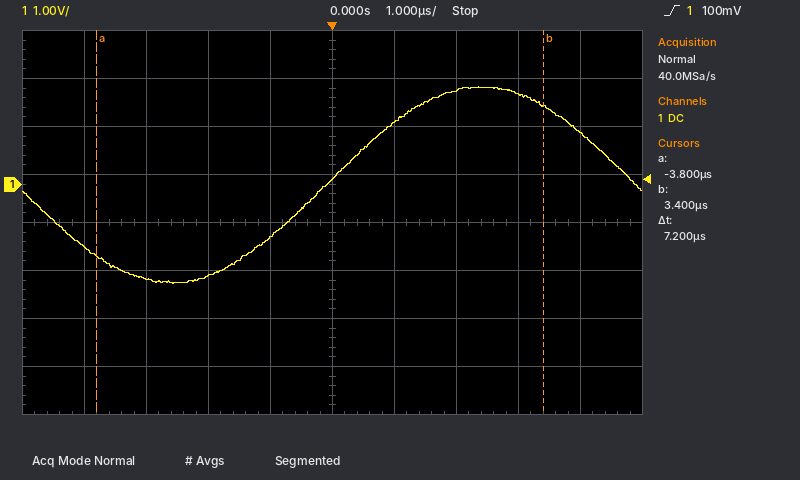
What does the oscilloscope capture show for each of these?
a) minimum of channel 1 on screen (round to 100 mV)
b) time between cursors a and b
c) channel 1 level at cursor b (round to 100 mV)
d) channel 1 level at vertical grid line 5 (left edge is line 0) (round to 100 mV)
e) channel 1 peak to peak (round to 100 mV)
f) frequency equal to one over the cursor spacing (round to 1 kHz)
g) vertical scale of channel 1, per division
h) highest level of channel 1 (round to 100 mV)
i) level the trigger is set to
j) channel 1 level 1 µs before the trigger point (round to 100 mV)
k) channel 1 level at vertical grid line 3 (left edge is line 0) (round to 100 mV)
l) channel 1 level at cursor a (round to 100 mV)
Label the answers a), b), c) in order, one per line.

a) -2.1 V
b) 7.2 µs
c) 1.6 V
d) 100 mV
e) 4.1 V
f) 139 kHz
g) 1 V
h) 2.0 V
i) 100 mV
j) -1.1 V
k) -1.9 V
l) -1.5 V
